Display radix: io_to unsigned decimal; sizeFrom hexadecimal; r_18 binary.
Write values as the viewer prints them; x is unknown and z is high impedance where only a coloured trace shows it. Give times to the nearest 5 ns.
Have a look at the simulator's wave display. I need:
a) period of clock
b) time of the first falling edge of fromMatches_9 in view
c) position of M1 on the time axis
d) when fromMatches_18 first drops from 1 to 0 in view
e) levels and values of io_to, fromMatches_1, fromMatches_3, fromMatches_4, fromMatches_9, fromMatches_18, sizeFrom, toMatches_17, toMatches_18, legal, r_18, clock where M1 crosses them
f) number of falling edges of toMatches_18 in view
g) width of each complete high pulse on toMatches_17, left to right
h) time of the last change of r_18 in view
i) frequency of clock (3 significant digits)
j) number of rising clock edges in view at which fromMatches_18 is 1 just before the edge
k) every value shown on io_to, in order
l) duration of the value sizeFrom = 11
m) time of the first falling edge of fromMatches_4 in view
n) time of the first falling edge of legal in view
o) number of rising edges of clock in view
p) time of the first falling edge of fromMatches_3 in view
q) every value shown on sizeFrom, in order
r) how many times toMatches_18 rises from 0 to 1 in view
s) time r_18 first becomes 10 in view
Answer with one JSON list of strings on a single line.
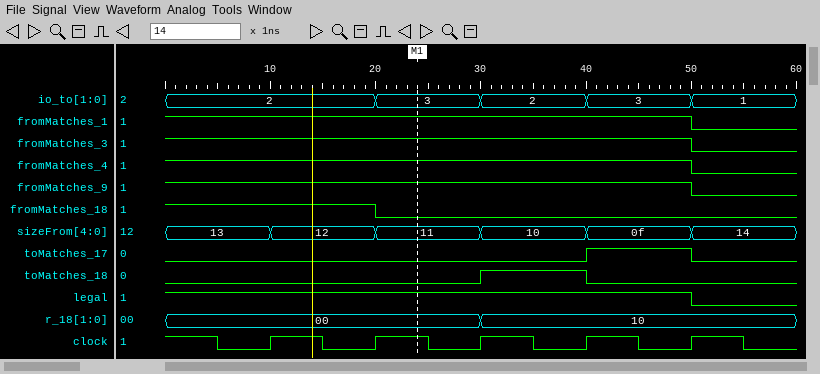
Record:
["10 ns", "50 ns", "25 ns", "20 ns", "io_to=3, fromMatches_1=1, fromMatches_3=1, fromMatches_4=1, fromMatches_9=1, fromMatches_18=0, sizeFrom=11, toMatches_17=0, toMatches_18=0, legal=1, r_18=00, clock=1", "1", "10 ns", "30 ns", "100 MHz", "2", "2, 3, 2, 3, 1", "10 ns", "50 ns", "50 ns", "5", "50 ns", "13, 12, 11, 10, 0f, 14", "1", "30 ns"]
